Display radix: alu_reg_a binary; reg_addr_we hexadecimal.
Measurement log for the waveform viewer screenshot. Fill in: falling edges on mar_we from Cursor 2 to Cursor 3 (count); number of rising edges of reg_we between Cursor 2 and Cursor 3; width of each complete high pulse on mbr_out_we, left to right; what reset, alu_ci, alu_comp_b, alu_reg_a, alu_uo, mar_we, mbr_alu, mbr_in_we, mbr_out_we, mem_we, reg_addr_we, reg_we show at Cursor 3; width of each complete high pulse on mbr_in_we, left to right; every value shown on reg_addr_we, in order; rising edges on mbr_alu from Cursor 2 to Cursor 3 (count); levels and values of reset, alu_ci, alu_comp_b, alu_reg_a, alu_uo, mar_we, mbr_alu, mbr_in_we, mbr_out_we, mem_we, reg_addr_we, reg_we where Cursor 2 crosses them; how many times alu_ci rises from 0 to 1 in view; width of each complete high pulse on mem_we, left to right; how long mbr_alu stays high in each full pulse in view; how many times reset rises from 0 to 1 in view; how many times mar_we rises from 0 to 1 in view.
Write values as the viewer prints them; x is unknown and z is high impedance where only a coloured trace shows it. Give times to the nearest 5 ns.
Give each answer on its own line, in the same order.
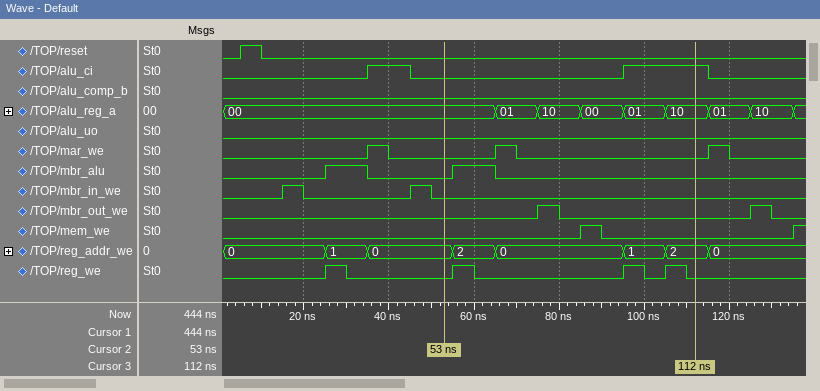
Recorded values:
1
3
5 ns, 5 ns
reset=0, alu_ci=1, alu_comp_b=0, alu_reg_a=10, alu_uo=0, mar_we=0, mbr_alu=0, mbr_in_we=0, mbr_out_we=0, mem_we=0, reg_addr_we=2, reg_we=0
5 ns, 5 ns
0, 1, 0, 2, 0, 1, 2, 0
1
reset=0, alu_ci=0, alu_comp_b=0, alu_reg_a=00, alu_uo=0, mar_we=0, mbr_alu=0, mbr_in_we=0, mbr_out_we=0, mem_we=0, reg_addr_we=0, reg_we=0
2
5 ns
10 ns, 10 ns
1
3
